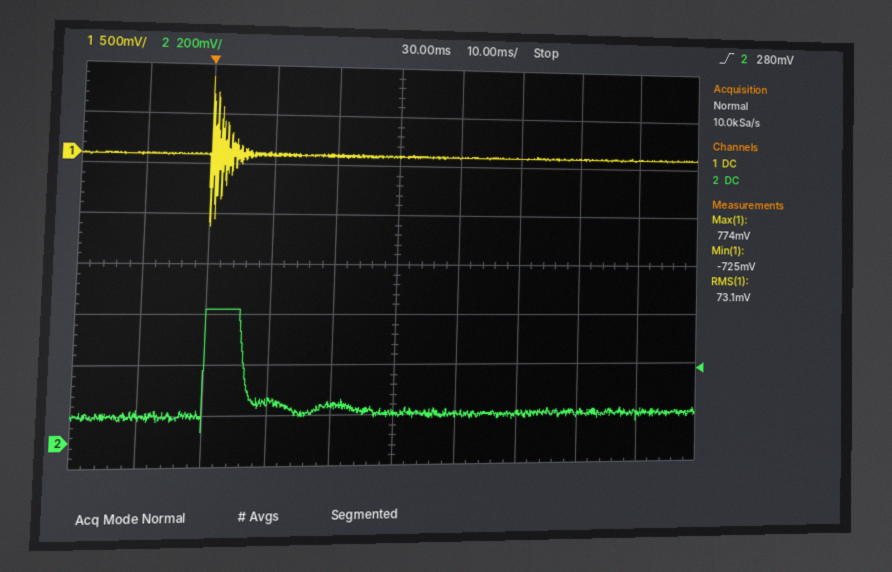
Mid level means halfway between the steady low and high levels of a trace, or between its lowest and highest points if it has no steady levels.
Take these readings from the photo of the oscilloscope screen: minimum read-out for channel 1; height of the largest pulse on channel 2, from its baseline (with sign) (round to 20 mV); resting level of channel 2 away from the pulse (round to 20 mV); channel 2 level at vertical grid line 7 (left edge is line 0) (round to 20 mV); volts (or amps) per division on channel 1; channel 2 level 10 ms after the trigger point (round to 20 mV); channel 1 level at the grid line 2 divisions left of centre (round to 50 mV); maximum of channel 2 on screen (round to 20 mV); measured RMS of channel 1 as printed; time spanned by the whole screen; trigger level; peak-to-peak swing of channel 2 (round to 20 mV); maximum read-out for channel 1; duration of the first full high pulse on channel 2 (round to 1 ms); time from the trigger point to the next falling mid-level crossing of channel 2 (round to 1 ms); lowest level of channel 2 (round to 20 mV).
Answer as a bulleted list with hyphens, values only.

- -725 mV
- +420 mV
- 100 mV
- 100 mV
- 500 mV
- 160 mV
- 0 mV
- 520 mV
- 73.1 mV
- 100 ms
- 280 mV
- 480 mV
- 774 mV
- 6 ms
- 6 ms
- 40 mV
